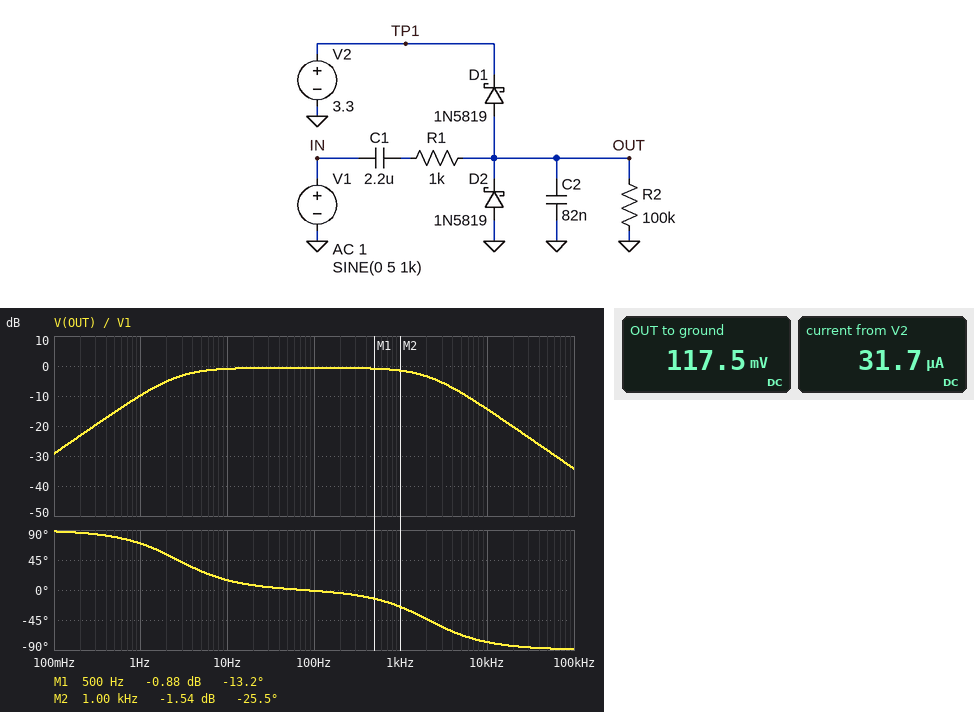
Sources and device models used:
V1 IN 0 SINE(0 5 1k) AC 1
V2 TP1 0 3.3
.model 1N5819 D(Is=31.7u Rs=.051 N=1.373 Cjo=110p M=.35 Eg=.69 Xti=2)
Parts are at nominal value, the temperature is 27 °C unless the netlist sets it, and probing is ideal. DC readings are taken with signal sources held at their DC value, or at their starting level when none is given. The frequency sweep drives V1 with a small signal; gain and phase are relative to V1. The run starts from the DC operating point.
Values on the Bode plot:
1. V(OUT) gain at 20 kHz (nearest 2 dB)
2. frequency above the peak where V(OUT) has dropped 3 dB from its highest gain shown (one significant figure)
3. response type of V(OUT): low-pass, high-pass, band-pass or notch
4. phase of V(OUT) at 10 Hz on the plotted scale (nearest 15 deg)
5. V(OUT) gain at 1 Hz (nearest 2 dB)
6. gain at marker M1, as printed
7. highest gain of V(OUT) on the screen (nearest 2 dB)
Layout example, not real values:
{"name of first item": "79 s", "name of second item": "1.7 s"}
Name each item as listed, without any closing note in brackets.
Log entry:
{"V(OUT) gain at 20 kHz": "-20 dB", "frequency above the peak where V(OUT) has dropped 3 dB from its highest gain shown": "2 kHz", "response type of V(OUT): low-pass, high-pass, band-pass or notch": "band-pass", "phase of V(OUT) at 10 Hz on the plotted scale": "15 deg", "V(OUT) gain at 1 Hz": "-10 dB", "gain at marker M1, as printed": "-0.88 dB", "highest gain of V(OUT) on the screen": "0 dB"}
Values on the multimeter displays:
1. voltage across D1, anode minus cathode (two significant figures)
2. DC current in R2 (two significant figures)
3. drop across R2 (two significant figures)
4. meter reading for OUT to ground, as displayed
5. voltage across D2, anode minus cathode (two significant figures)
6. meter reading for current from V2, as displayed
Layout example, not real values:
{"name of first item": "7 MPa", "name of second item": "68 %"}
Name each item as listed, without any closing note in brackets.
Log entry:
{"voltage across D1, anode minus cathode": "-3.2 V", "DC current in R2": "1.2 µA", "drop across R2": "120 mV", "meter reading for OUT to ground, as displayed": "117.5 mV", "voltage across D2, anode minus cathode": "-120 mV", "meter reading for current from V2, as displayed": "31.7 µA"}
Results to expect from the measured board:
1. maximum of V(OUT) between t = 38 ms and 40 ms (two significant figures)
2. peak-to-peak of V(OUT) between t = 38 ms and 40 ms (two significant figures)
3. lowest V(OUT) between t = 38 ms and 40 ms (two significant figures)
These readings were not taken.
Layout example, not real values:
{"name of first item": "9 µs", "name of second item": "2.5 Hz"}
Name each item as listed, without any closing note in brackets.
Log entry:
{"maximum of V(OUT) between t = 38 ms and 40 ms": "3.5 V", "peak-to-peak of V(OUT) between t = 38 ms and 40 ms": "3.6 V", "lowest V(OUT) between t = 38 ms and 40 ms": "-160 mV"}
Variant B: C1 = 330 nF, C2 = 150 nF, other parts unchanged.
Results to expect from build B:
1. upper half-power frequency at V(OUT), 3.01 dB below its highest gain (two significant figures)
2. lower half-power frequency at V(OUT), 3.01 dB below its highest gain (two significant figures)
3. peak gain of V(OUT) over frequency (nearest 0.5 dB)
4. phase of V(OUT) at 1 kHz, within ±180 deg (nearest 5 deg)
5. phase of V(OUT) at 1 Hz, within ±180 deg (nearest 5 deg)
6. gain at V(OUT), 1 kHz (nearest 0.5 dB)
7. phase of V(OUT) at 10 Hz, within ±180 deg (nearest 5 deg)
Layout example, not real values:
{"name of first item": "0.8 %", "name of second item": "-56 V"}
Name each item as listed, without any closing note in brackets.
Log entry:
{"upper half-power frequency at V(OUT), 3.01 dB below its highest gain": "1.6 kHz", "lower half-power frequency at V(OUT), 3.01 dB below its highest gain": "13 Hz", "peak gain of V(OUT) over frequency": "-3.5 dB", "phase of V(OUT) at 1 kHz, within ±180 deg": "-30 deg", "phase of V(OUT) at 1 Hz, within ±180 deg": "85 deg", "gain at V(OUT), 1 kHz": "-5.0 dB", "phase of V(OUT) at 10 Hz, within ±180 deg": "50 deg"}
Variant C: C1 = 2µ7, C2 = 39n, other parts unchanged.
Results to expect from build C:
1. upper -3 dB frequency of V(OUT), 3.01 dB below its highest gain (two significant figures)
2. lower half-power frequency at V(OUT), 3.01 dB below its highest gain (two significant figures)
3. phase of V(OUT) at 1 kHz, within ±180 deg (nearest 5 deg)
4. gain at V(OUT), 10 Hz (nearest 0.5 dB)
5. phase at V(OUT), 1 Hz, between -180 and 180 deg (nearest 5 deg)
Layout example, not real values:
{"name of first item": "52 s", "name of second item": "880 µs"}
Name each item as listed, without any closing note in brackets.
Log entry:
{"upper -3 dB frequency of V(OUT), 3.01 dB below its highest gain": "4.3 kHz", "lower half-power frequency at V(OUT), 3.01 dB below its highest gain": "2.2 Hz", "phase of V(OUT) at 1 kHz, within ±180 deg": "-15 deg", "gain at V(OUT), 10 Hz": "-0.5 dB", "phase at V(OUT), 1 Hz, between -180 and 180 deg": "65 deg"}
